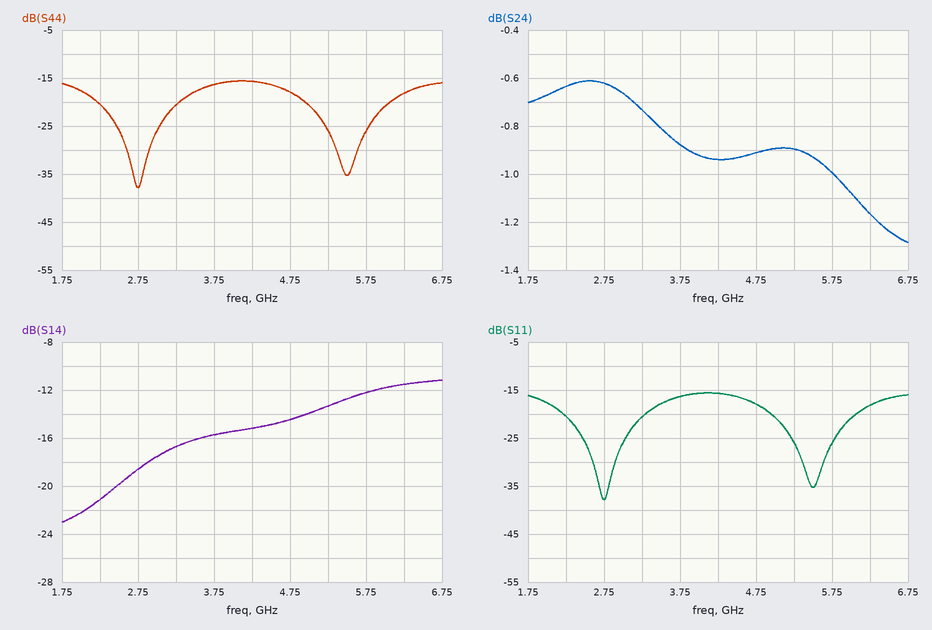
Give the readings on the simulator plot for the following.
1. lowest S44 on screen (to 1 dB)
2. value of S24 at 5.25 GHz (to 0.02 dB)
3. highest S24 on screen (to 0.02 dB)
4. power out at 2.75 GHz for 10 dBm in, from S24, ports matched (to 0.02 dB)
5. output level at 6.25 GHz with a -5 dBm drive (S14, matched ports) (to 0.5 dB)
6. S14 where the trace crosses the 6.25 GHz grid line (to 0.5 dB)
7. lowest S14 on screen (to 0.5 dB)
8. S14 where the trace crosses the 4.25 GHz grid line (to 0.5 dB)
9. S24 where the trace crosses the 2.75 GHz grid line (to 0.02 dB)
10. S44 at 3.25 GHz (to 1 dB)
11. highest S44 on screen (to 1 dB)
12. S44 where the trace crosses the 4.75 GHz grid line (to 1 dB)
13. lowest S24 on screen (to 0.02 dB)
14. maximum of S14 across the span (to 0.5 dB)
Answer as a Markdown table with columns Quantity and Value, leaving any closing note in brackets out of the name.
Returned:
| Quantity | Value |
|---|---|
| lowest S44 on screen | -38 dB |
| value of S24 at 5.25 GHz | -0.90 dB |
| highest S24 on screen | -0.62 dB |
| power out at 2.75 GHz for 10 dBm in, from S24, ports matched | 9.38 dBm |
| output level at 6.25 GHz with a -5 dBm drive (S14, matched ports) | -16.5 dBm |
| S14 where the trace crosses the 6.25 GHz grid line | -11.5 dB |
| lowest S14 on screen | -23.0 dB |
| S14 where the trace crosses the 4.25 GHz grid line | -15.0 dB |
| S24 where the trace crosses the 2.75 GHz grid line | -0.62 dB |
| S44 at 3.25 GHz | -21 dB |
| highest S44 on screen | -16 dB |
| S44 where the trace crosses the 4.75 GHz grid line | -18 dB |
| lowest S24 on screen | -1.28 dB |
| maximum of S14 across the span | -11.0 dB |
